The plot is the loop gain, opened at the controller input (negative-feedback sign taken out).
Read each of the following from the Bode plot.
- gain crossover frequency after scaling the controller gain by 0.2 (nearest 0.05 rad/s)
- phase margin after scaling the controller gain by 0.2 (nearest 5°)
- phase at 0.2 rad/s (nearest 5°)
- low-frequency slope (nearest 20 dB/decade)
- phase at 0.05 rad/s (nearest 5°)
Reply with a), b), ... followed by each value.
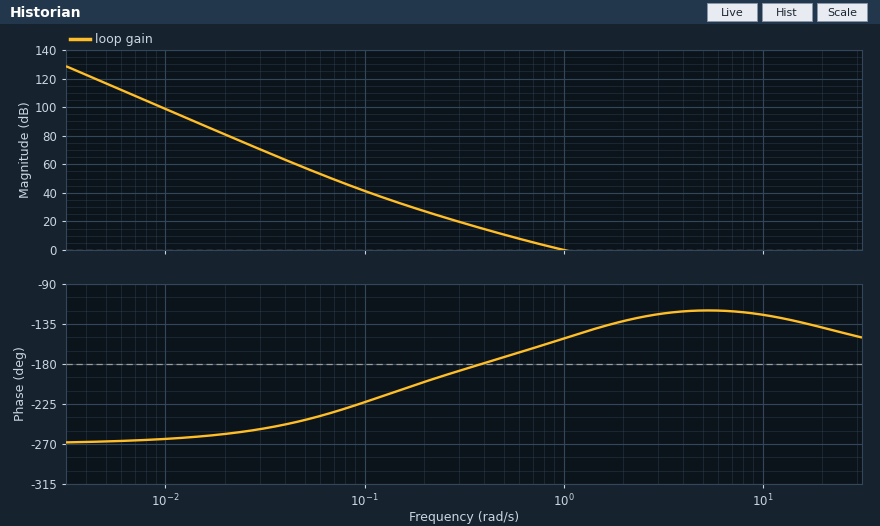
a) 0.40 rad/s
b) 0°
c) -200°
d) -60 dB/decade
e) -245°
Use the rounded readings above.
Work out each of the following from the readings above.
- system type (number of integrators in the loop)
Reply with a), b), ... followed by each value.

a) 3
